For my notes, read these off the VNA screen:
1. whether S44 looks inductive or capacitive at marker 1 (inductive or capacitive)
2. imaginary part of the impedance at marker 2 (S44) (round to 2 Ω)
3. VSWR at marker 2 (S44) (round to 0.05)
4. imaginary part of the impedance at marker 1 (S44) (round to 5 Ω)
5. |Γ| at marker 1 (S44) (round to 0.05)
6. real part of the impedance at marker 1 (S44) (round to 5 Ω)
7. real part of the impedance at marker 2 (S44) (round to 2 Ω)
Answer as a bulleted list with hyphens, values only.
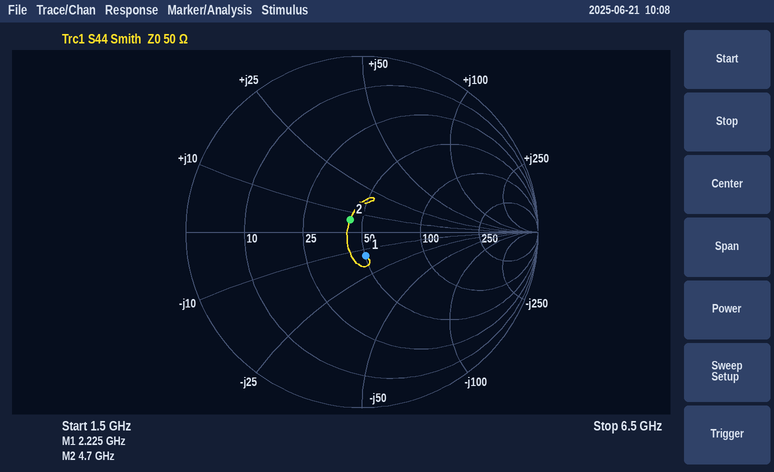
- capacitive
- +6 Ω
- 1.20
- -15 Ω
- 0.15
- 50 Ω
- 44 Ω
